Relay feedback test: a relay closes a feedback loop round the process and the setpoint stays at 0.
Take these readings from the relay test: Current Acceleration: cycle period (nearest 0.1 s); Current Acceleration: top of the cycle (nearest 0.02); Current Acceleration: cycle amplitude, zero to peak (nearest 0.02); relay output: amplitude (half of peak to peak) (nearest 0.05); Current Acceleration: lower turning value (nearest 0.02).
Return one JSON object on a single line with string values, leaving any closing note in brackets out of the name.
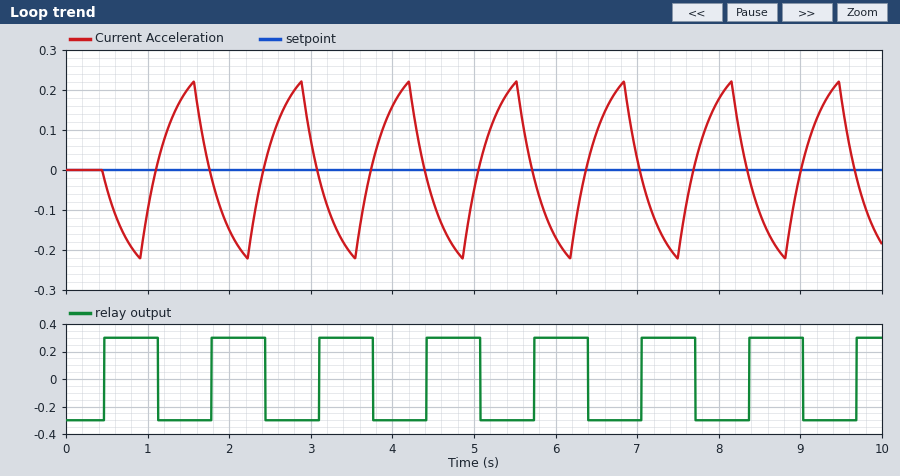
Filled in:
{"Current Acceleration: cycle period": "1.3 s", "Current Acceleration: top of the cycle": "0.22", "Current Acceleration: cycle amplitude, zero to peak": "0.22", "relay output: amplitude (half of peak to peak)": "0.30", "Current Acceleration: lower turning value": "-0.22"}
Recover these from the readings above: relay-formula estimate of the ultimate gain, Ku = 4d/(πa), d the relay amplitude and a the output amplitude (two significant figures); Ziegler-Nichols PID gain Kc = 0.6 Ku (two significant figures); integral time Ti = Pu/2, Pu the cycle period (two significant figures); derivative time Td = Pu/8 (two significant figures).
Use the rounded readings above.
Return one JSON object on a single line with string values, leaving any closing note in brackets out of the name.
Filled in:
{"relay-formula estimate of the ultimate gain, Ku = 4d/(πa), d the relay amplitude and a the output amplitude": "1.7", "Ziegler-Nichols PID gain Kc = 0.6 Ku": "1.0", "integral time Ti = Pu/2, Pu the cycle period": "0.65 s", "derivative time Td = Pu/8": "0.16 s"}
